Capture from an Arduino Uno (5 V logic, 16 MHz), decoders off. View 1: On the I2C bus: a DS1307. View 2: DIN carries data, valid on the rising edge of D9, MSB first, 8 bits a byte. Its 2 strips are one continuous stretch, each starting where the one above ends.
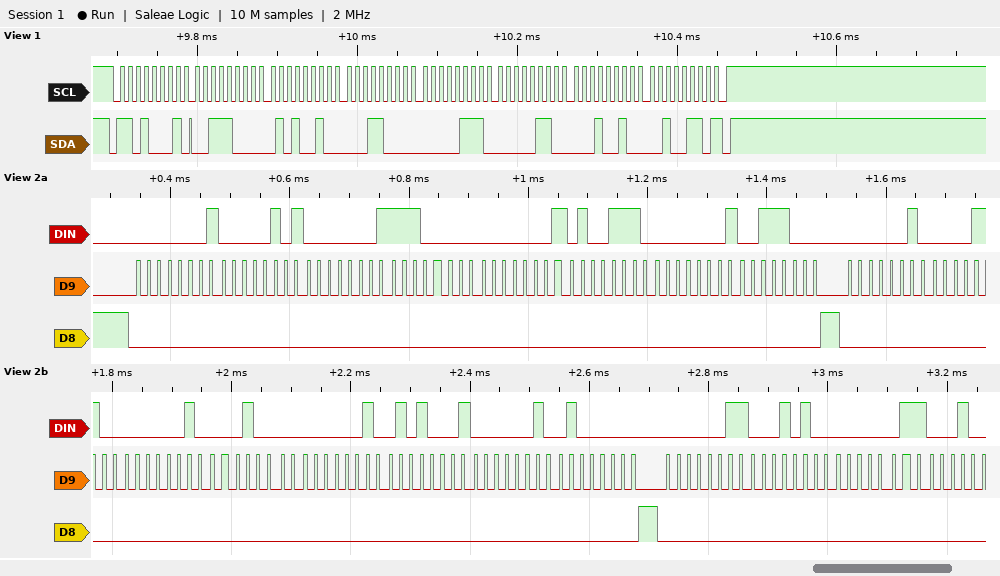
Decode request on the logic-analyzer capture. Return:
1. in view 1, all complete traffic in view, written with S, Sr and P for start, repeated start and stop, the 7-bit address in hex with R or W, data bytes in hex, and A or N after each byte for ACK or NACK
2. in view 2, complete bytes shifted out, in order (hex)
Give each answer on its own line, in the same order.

S 68R A 38 A 52 A 18 A 07 A 06 A 12 A 26 N P
01 05 01 E0 01 4E 01 38 02 0C 02 10 02 51 02 40 03 14 03
